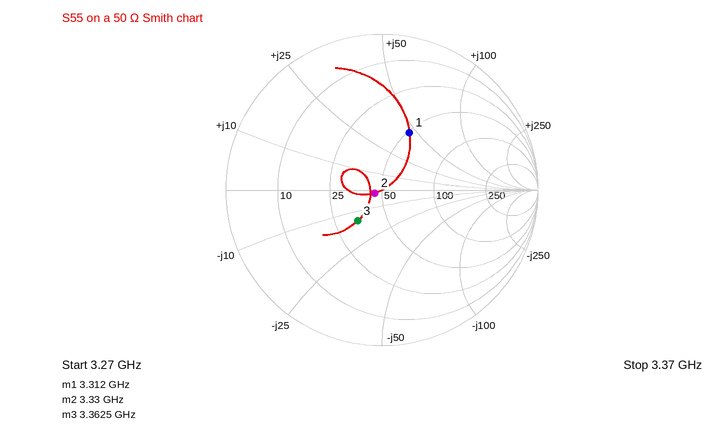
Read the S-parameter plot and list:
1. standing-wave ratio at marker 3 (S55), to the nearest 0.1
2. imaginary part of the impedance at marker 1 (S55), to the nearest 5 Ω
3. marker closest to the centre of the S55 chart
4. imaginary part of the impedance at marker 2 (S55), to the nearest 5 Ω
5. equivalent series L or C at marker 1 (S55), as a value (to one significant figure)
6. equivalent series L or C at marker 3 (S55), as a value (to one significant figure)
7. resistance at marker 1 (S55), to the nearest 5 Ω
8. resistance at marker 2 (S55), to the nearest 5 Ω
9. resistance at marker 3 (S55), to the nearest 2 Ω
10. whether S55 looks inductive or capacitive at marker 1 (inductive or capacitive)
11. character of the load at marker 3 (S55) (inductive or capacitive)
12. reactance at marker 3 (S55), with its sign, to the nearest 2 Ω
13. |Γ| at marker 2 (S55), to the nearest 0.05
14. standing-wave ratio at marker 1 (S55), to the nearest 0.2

1.7
+45 Ω
marker 2
0 Ω
2 nH
3 pF
50 Ω
45 Ω
34 Ω
inductive
capacitive
-14 Ω
0.05
2.4
